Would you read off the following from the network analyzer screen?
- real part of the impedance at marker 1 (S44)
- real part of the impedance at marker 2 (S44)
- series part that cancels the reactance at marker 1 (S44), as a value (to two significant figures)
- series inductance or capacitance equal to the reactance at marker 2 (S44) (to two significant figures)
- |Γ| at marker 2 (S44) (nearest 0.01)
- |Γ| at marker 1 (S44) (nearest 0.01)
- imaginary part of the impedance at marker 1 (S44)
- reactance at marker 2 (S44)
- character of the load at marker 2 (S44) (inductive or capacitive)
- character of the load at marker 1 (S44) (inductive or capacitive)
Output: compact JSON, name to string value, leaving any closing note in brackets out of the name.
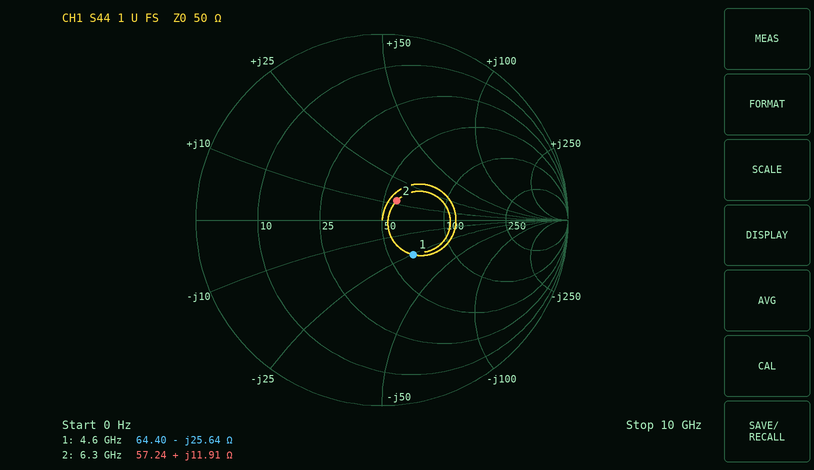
{"real part of the impedance at marker 1": "64.40 Ω", "real part of the impedance at marker 2": "57.24 Ω", "series part that cancels the reactance at marker 1 (S44), as a value": "890 pH", "series inductance or capacitance equal to the reactance at marker 2 (S44)": "300 pH", "|Γ| at marker 2 (S44)": "0.13", "|Γ| at marker 1 (S44)": "0.25", "imaginary part of the impedance at marker 1": "-25.64 Ω", "reactance at marker 2": "+11.91 Ω", "character of the load at marker 2 (S44)": "inductive", "character of the load at marker 1 (S44)": "capacitive"}
